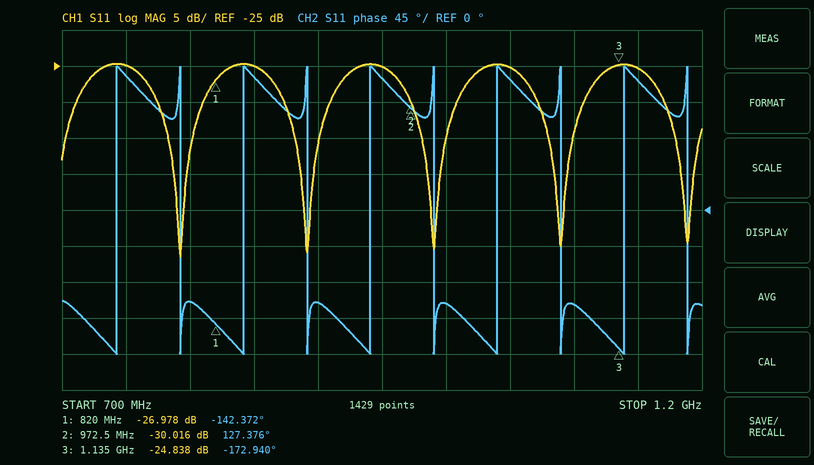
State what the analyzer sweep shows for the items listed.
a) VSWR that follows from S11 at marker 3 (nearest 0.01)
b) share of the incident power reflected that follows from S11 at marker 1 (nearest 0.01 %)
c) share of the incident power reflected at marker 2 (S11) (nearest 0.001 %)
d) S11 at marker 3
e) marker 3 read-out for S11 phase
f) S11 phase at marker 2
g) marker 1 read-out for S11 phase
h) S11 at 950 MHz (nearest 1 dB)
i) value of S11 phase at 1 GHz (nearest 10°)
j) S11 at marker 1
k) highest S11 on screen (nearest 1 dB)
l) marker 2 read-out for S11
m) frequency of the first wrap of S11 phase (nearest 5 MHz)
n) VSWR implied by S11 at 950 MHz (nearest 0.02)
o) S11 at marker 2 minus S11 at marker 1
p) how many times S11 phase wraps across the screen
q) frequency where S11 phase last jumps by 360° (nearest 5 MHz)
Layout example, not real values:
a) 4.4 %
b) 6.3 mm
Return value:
a) 1.12
b) 0.20 %
c) 0.100 %
d) -24.838 dB
e) -172.940°
f) 127.376°
g) -142.372°
h) -25 dB
i) -120°
j) -26.978 dB
k) -25 dB
l) -30.016 dB
m) 745 MHz
n) 1.12
o) -3.038 dB
p) 10
q) 1.190 GHz
